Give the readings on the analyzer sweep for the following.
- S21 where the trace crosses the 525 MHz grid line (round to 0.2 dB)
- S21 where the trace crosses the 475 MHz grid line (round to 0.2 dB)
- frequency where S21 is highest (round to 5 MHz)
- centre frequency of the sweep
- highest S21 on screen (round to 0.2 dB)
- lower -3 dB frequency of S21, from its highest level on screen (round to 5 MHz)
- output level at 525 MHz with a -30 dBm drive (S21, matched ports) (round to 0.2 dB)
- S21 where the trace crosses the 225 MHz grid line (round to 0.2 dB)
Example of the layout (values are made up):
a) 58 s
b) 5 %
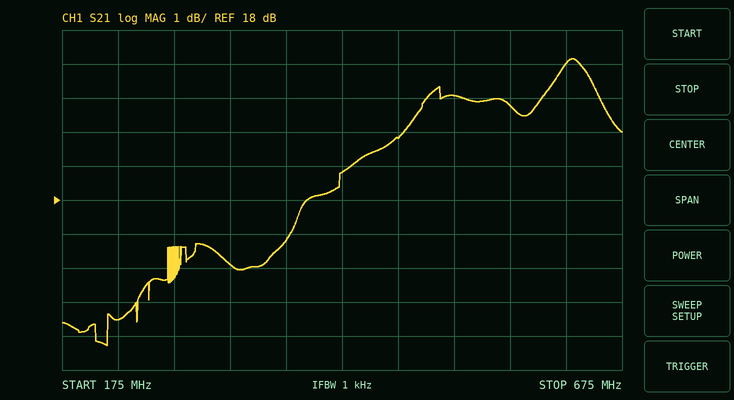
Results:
a) 21.0 dB
b) 19.8 dB
c) 630 MHz
d) 425 MHz
e) 22.2 dB
f) 440 MHz
g) -9.0 dBm
h) 14.4 dB
